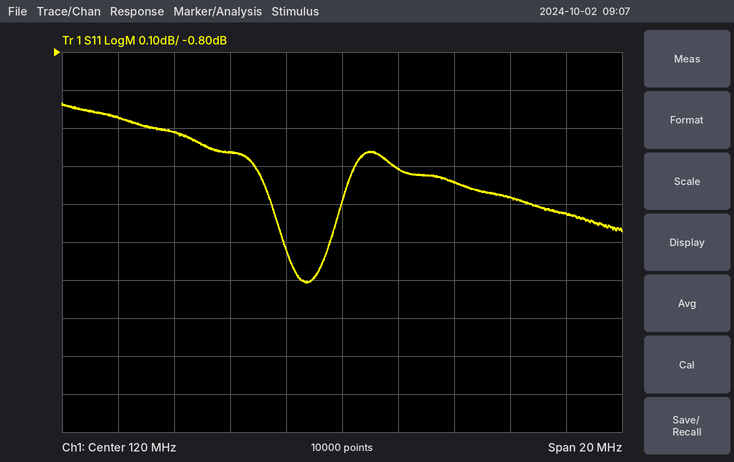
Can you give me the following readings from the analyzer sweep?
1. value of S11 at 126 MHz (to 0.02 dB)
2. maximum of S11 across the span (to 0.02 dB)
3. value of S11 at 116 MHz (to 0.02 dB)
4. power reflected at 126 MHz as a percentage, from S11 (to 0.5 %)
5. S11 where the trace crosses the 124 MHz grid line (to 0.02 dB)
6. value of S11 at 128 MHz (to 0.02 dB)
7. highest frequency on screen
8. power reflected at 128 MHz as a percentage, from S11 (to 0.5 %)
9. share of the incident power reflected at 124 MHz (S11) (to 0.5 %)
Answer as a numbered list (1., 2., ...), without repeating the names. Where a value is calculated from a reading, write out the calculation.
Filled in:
1. -1.18 dB
2. -0.94 dB
3. -1.06 dB
4. 10^(-1.18/10) ≈ 76.2 %, so 76.0 % to the nearest 0.5 %
5. -1.14 dB
6. -1.22 dB
7. 130 MHz
8. 10^(-1.22/10) ≈ 75.5 %
9. 10^(-1.14/10) ≈ 76.9 %, so 77.0 % to the nearest 0.5 %
